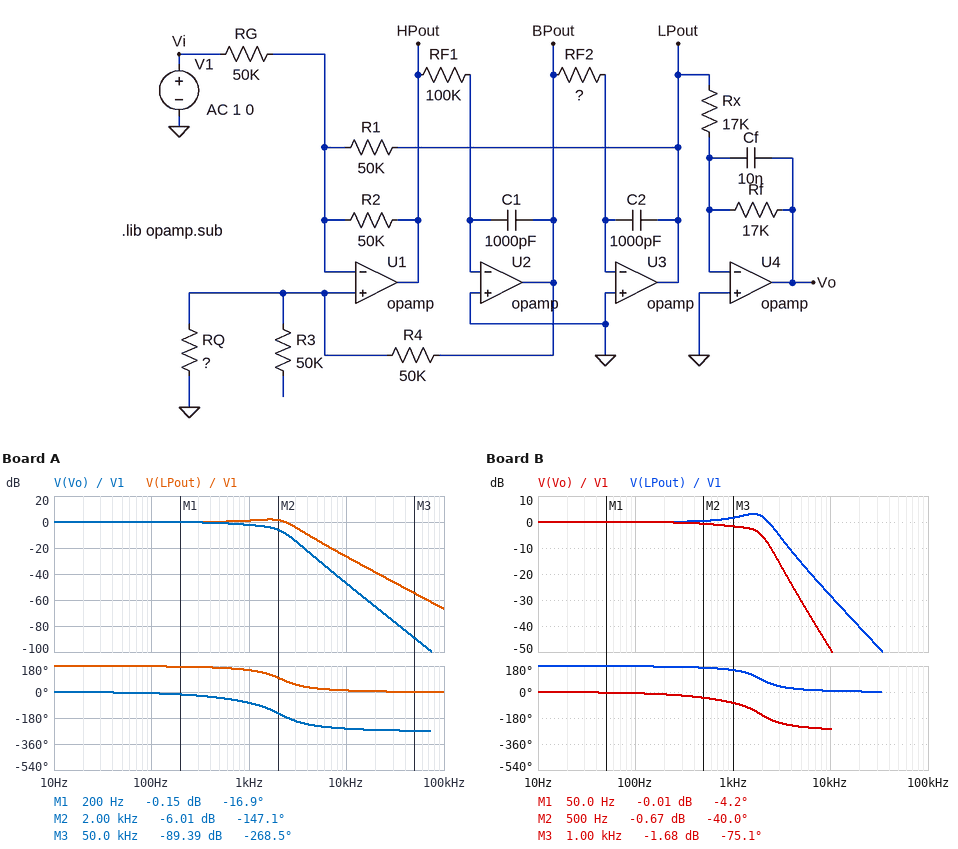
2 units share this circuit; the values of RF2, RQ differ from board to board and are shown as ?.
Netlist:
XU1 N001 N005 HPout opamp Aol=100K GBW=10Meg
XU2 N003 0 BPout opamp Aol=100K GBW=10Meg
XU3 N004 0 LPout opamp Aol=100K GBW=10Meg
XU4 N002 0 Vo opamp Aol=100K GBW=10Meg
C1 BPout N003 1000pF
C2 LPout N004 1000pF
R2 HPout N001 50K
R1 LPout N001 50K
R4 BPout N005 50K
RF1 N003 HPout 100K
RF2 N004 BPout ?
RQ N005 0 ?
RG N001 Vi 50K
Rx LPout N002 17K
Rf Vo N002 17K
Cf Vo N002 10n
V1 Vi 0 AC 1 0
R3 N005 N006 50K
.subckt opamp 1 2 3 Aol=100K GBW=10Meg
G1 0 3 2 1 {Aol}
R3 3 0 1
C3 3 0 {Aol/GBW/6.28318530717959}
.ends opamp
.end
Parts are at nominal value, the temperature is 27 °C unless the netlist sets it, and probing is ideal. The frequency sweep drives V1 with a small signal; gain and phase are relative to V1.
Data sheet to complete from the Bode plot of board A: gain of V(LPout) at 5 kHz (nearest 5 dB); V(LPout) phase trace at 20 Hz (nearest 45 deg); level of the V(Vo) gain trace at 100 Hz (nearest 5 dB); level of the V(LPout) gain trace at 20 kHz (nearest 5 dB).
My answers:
-15 dB
180 deg
0 dB
-40 dB
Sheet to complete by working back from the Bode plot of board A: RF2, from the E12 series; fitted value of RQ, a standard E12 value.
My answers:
56 kΩ
33 kΩ
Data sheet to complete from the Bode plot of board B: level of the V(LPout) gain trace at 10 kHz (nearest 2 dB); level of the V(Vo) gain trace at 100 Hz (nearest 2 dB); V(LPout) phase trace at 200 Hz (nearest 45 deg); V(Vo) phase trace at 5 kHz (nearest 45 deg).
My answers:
-28 dB
0 dB
180 deg
-225 deg
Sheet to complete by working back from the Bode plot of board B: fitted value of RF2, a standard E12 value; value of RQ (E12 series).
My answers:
68 kΩ
22 kΩ
